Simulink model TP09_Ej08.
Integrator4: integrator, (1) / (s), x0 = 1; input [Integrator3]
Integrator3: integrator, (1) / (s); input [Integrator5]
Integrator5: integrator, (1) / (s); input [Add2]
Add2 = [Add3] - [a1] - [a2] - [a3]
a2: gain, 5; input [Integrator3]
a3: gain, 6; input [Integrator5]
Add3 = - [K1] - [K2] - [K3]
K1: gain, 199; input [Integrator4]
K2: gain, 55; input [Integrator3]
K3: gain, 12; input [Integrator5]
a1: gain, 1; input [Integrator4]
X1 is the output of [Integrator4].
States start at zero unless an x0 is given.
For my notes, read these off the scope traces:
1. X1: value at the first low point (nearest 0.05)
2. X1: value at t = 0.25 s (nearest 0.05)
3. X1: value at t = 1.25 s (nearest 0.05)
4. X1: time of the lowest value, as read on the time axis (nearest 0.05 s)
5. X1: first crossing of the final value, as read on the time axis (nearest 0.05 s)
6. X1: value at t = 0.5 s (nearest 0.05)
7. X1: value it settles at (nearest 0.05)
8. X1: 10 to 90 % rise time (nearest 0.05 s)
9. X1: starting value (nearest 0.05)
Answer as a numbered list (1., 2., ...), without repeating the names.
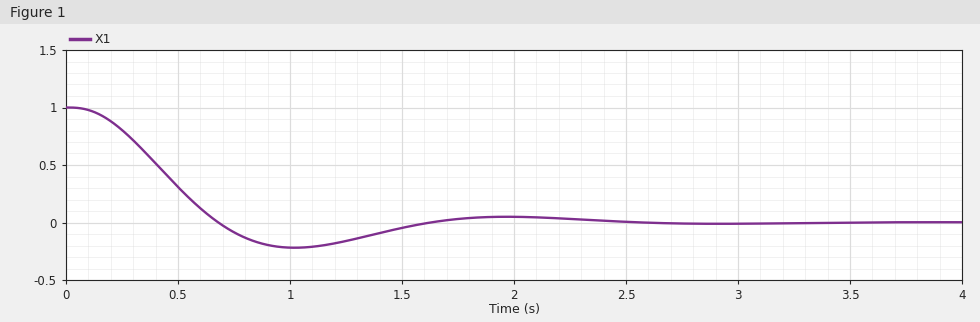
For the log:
1. -0.20
2. 0.80
3. -0.15
4. 1.00 s
5. 0.70 s
6. 0.30
7. 0.00
8. 0.45 s
9. 1.00
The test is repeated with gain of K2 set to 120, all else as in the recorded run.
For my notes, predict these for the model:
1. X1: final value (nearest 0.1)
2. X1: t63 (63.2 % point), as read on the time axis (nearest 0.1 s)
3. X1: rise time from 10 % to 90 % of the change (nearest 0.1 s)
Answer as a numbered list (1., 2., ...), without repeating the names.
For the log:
1. 0.0
2. 0.6 s
3. 1.0 s
